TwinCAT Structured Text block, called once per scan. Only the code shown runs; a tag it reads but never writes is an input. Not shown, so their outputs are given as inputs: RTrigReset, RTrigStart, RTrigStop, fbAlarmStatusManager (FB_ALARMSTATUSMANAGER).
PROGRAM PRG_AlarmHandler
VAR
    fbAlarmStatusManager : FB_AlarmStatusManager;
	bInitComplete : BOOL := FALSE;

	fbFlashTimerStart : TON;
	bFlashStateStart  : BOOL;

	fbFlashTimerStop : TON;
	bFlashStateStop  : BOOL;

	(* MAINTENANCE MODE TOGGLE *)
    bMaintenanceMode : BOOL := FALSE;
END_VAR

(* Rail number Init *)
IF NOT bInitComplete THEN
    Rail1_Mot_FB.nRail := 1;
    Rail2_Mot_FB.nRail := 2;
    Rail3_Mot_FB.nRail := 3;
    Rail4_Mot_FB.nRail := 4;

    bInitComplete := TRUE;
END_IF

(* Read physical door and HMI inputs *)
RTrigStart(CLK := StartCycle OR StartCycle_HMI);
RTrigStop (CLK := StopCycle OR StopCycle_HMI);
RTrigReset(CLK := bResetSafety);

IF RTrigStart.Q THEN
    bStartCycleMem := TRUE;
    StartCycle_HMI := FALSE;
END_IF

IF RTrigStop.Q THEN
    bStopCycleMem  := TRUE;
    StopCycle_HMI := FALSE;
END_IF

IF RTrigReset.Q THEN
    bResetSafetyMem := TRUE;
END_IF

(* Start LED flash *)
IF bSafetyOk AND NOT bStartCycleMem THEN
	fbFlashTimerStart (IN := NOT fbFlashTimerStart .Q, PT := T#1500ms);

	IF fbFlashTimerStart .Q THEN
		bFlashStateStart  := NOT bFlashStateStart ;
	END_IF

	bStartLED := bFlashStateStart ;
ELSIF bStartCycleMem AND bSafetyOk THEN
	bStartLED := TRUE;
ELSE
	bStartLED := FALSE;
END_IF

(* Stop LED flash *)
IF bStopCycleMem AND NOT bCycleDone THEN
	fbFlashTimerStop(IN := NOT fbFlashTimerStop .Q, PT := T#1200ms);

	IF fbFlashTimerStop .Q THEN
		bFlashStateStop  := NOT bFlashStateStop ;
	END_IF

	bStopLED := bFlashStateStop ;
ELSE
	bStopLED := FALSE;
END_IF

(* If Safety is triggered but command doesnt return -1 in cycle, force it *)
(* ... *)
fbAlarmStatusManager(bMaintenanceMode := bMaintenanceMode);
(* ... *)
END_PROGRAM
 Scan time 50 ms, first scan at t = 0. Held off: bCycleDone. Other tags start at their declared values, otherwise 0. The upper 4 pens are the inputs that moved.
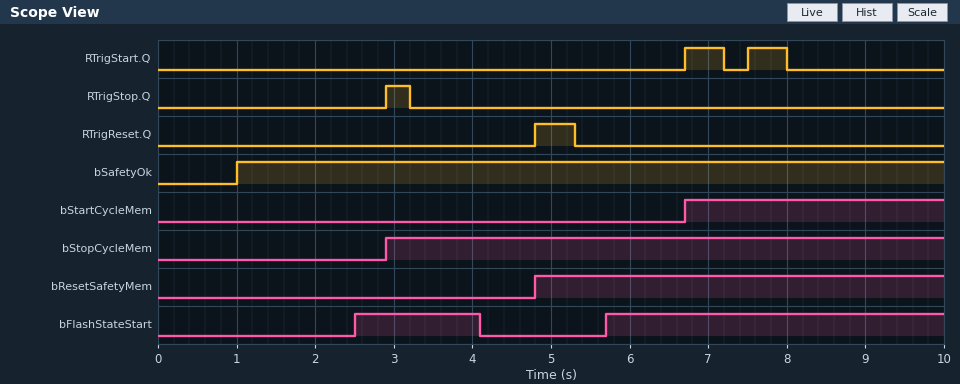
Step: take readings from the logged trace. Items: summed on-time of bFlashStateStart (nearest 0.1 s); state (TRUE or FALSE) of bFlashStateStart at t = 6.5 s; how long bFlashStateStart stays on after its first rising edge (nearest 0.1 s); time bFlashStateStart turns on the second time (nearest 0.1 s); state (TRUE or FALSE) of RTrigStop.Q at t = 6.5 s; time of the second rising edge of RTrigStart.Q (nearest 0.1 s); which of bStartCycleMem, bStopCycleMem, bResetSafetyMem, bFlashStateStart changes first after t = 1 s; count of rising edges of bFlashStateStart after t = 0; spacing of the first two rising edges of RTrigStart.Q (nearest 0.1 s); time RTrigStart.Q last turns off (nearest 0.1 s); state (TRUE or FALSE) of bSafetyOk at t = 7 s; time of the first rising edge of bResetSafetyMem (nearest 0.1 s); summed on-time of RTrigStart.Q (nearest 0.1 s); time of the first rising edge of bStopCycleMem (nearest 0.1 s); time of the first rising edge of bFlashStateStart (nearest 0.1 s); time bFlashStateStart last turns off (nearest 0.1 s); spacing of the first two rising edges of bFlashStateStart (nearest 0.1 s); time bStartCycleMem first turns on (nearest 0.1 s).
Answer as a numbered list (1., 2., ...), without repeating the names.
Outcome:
1. 5.9 s
2. TRUE
3. 1.6 s
4. 5.7 s
5. FALSE
6. 7.5 s
7. bFlashStateStart
8. 2
9. 0.8 s
10. 8.0 s
11. TRUE
12. 4.8 s
13. 1.0 s
14. 2.9 s
15. 2.5 s
16. 4.1 s
17. 3.2 s
18. 6.7 s
